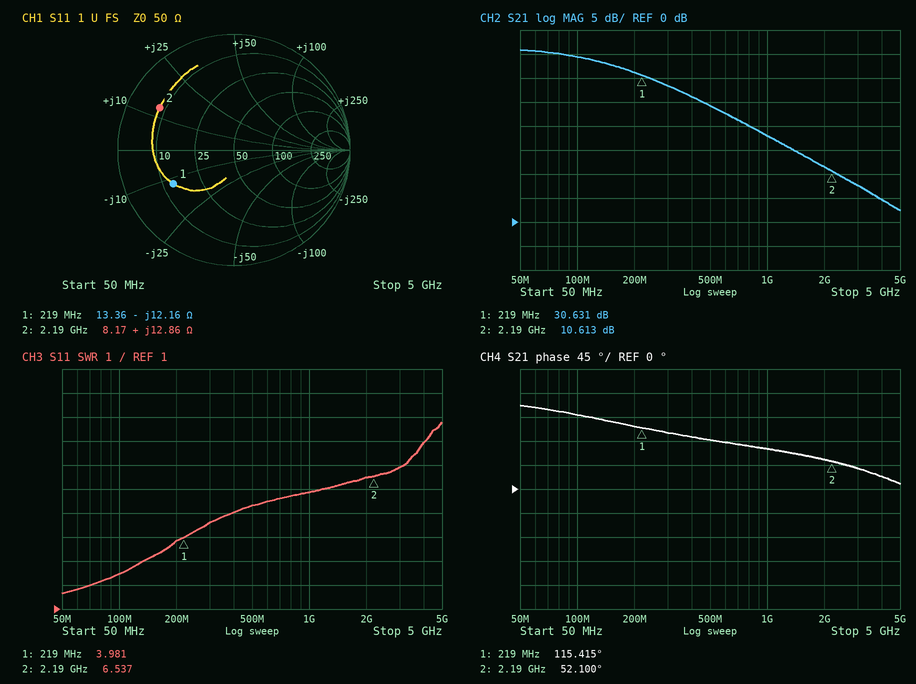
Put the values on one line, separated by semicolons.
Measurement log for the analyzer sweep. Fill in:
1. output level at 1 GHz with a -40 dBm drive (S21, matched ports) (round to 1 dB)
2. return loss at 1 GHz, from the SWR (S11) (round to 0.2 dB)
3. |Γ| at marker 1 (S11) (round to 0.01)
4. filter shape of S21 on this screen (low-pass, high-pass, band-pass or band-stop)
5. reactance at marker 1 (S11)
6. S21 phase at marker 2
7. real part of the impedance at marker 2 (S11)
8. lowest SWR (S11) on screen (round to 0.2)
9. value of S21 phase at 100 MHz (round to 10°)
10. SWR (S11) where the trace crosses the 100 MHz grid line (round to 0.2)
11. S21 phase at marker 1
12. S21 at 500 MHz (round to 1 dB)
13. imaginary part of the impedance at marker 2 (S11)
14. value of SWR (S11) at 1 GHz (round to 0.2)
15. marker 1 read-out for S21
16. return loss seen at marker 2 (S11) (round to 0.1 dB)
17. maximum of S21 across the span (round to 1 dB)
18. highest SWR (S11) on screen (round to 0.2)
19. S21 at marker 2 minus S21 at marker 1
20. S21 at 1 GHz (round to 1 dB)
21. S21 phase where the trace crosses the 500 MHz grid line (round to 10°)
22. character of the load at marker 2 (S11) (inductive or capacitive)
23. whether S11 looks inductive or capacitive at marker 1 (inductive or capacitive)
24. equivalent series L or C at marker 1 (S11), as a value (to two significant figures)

-22 dBm; 3.0 dB; 0.60; low-pass; -12.16 Ω; 52.100°; 8.17 Ω; 1.6; 140°; 2.4; 115.415°; 24 dB; +12.86 Ω; 5.8; 30.631 dB; 2.7 dB; 36 dB; 8.8; -20.018 dB; 18 dB; 90°; inductive; capacitive; 60 pF
